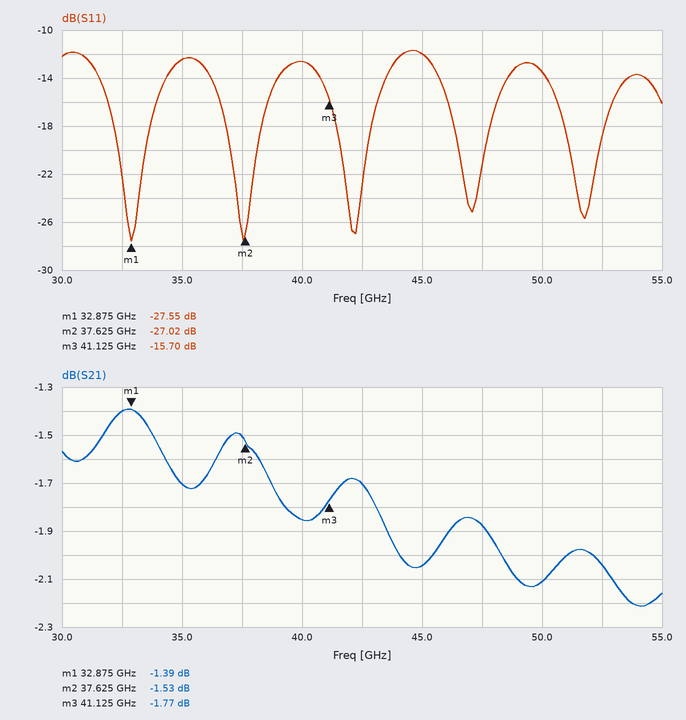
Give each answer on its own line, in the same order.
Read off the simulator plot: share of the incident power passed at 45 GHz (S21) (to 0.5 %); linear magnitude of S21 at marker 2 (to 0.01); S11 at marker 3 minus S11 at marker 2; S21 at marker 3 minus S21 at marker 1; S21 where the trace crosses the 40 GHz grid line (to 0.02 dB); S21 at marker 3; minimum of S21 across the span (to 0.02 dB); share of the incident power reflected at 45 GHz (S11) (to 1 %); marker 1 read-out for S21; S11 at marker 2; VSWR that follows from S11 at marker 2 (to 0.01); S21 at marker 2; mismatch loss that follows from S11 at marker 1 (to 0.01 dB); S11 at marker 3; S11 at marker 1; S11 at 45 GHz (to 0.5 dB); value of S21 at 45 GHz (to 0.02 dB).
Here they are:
62.5 %
0.84
11.32 dB
-0.38 dB
-1.86 dB
-1.77 dB
-2.22 dB
6 %
-1.39 dB
-27.02 dB
1.09
-1.53 dB
0.01 dB
-15.70 dB
-27.55 dB
-12.0 dB
-2.04 dB
